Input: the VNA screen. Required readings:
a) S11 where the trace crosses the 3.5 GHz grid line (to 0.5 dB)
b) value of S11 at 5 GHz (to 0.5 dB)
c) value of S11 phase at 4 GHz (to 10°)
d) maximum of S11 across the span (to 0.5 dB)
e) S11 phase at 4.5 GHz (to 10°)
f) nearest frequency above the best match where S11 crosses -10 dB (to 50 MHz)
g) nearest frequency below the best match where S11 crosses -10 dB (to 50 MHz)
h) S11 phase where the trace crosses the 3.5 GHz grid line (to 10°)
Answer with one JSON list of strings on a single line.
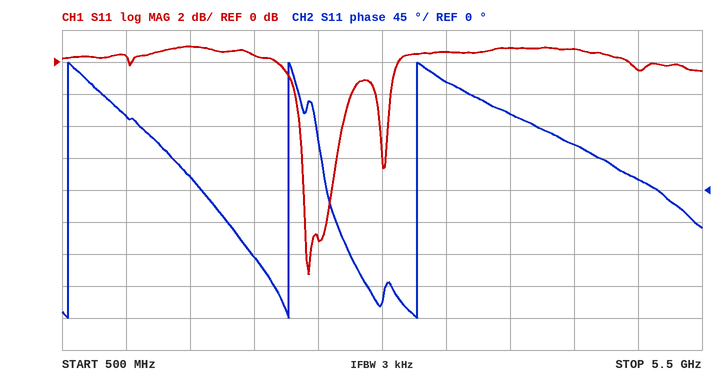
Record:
["0.5 dB", "-0.5 dB", "110°", "1.0 dB", "60°", "2.55 GHz", "2.40 GHz", "150°"]
